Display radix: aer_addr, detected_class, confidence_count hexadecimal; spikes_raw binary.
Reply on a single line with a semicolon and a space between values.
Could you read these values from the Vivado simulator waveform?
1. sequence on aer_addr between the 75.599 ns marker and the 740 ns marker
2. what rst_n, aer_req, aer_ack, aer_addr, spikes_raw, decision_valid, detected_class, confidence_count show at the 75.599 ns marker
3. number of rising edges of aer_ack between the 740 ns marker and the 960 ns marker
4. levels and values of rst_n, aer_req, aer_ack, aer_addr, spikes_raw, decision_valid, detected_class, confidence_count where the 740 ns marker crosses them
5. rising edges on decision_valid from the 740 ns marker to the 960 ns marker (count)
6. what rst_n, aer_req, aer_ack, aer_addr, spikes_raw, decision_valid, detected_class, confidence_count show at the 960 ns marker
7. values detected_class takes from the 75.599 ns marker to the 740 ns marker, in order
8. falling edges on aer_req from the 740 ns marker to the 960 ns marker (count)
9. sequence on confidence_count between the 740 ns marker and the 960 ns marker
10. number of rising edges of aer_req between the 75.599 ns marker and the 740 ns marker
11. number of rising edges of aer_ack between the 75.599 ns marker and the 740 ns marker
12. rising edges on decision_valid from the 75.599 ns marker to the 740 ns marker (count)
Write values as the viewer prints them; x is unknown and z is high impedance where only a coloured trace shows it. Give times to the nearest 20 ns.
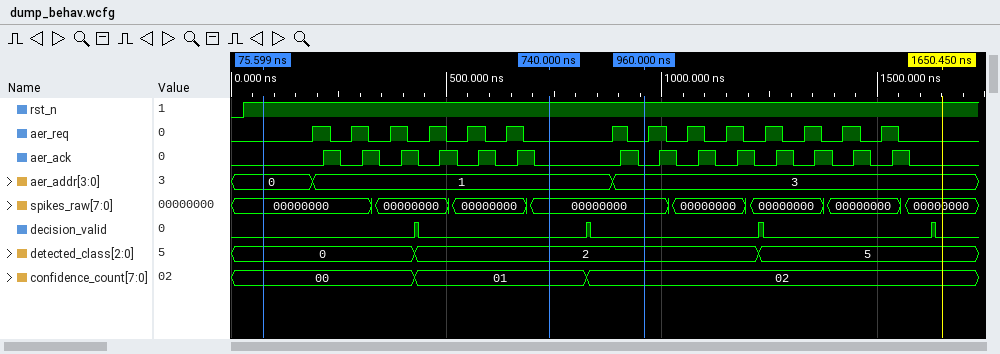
0, 1; rst_n=1, aer_req=0, aer_ack=0, aer_addr=0, spikes_raw=00000000, decision_valid=0, detected_class=0, confidence_count=00; 1; rst_n=1, aer_req=0, aer_ack=0, aer_addr=1, spikes_raw=00000000, decision_valid=0, detected_class=2, confidence_count=01; 1; rst_n=1, aer_req=0, aer_ack=0, aer_addr=3, spikes_raw=00000000, decision_valid=0, detected_class=2, confidence_count=02; 0, 2; 1; 01, 02; 6; 6; 1
